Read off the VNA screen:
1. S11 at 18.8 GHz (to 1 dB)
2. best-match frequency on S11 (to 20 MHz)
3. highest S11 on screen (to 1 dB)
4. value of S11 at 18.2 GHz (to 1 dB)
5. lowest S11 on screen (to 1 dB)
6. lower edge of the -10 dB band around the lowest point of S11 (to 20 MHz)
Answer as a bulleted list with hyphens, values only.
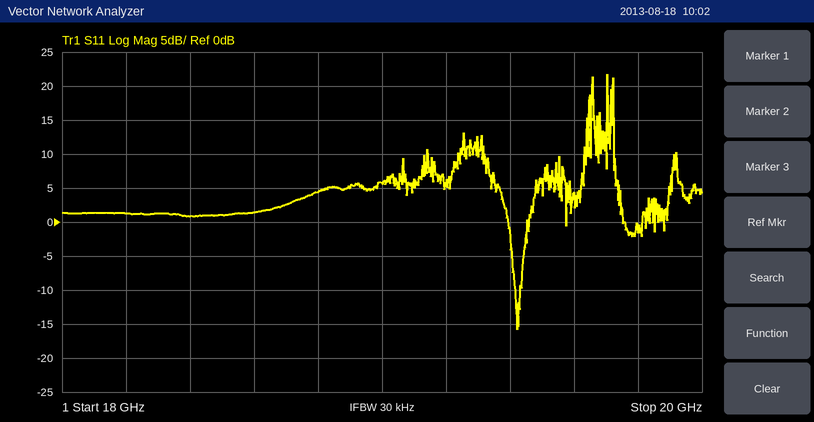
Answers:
- 4 dB
- 19.42 GHz
- 22 dB
- 1 dB
- -16 dB
- 19.42 GHz
